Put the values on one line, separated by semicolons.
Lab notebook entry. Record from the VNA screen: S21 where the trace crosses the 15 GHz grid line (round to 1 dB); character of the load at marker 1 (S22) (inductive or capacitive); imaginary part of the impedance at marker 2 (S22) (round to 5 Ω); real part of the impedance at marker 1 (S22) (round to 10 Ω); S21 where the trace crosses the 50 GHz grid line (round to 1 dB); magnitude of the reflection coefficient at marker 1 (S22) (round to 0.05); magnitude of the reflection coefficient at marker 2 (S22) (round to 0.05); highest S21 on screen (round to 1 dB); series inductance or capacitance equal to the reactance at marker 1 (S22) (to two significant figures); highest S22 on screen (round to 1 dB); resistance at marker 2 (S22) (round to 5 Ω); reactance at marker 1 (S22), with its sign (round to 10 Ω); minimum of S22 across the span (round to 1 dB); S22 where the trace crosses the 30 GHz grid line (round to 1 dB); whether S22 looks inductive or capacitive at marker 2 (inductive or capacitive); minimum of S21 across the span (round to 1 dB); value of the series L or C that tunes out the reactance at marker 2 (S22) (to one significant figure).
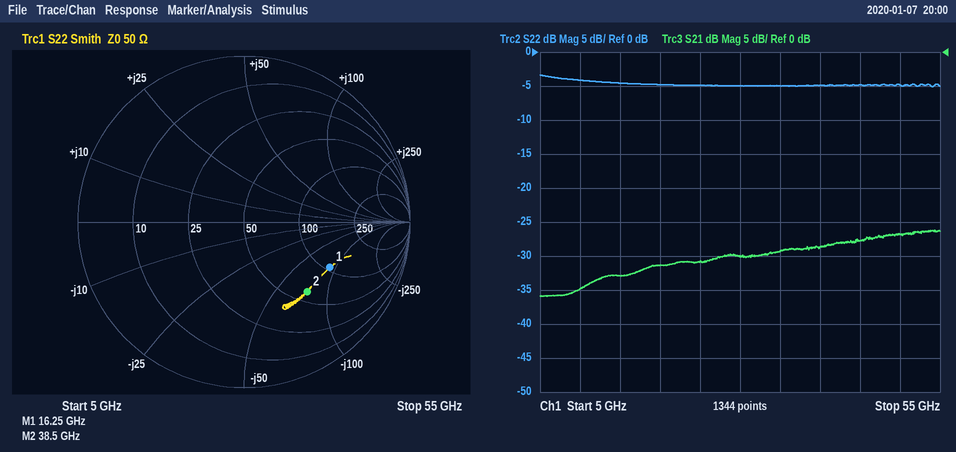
-33 dB; capacitive; -75 Ω; 110 Ω; -27 dB; 0.60; 0.55; -26 dB; 110 fF; -3 dB; 60 Ω; -90 Ω; -5 dB; -5 dB; capacitive; -36 dB; 300 pH
